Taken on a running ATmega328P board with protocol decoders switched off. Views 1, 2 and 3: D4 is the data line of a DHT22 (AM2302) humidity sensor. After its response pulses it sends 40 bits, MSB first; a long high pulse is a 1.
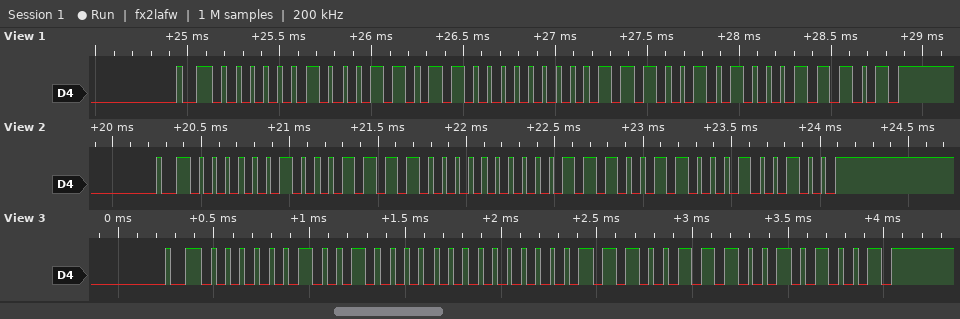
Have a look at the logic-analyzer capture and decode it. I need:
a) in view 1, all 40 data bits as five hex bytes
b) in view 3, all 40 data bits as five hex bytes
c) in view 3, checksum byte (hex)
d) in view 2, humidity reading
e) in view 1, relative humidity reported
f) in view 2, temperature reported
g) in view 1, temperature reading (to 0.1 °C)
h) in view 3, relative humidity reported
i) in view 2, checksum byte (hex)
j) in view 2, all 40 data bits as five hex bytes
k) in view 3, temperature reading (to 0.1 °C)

02 36 00 E5 1D
02 40 00 E7 29
0x29
57.2 %
56.6 %
23.0 °C
22.9 °C
57.6 %
0x24
02 3C 00 E6 24
23.1 °C
